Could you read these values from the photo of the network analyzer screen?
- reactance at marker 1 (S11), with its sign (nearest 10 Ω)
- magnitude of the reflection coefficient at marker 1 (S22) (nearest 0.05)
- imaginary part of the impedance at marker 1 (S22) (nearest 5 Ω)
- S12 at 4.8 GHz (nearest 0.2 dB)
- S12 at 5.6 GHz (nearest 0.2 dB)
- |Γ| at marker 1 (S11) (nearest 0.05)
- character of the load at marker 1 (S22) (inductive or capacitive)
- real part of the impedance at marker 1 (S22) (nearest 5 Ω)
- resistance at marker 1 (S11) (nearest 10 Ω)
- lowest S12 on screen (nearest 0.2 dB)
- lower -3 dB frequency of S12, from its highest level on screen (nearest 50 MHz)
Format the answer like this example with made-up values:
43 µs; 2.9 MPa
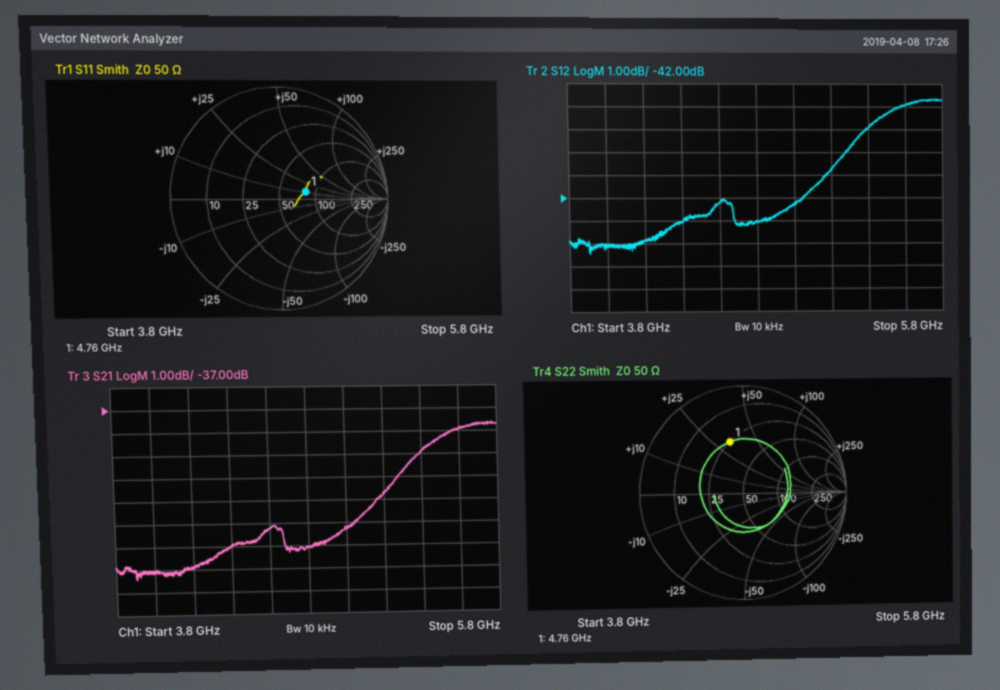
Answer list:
+10 Ω; 0.50; +30 Ω; -43.0 dB; -38.0 dB; 0.25; inductive; 25 Ω; 80 Ω; -44.4 dB; 5.20 GHz
